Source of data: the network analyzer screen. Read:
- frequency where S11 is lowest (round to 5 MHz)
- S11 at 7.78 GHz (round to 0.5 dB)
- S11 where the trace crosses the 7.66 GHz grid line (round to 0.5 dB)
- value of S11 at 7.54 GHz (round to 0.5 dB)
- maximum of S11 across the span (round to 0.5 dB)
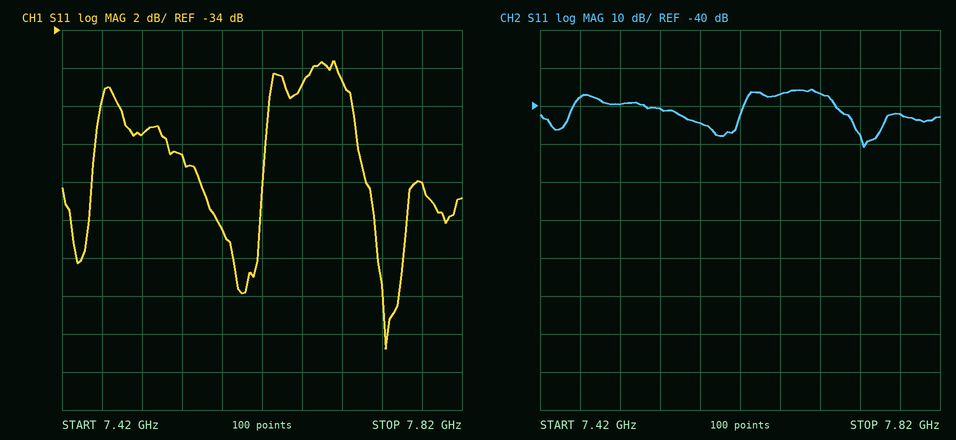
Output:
7.745 GHz
-42.0 dB
-37.0 dB
-40.5 dB
-35.5 dB
